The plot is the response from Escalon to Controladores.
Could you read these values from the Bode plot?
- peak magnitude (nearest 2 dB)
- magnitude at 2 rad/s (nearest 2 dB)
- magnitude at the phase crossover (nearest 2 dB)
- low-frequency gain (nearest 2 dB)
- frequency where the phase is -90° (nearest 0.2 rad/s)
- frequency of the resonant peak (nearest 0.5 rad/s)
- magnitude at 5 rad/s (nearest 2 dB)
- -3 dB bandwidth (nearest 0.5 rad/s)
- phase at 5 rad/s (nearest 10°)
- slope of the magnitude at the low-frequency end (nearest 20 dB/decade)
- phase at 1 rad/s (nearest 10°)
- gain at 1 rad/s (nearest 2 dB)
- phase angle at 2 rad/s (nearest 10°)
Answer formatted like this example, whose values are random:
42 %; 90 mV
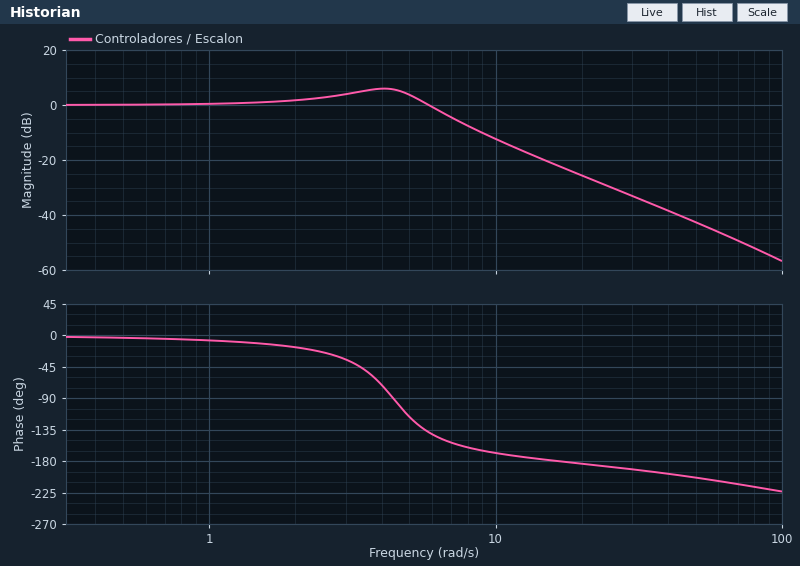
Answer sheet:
6 dB; 2 dB; -22 dB; 0 dB; 4.4 rad/s; 4.0 rad/s; 4 dB; 6.5 rad/s; -120°; 0 dB/decade; -10°; 0 dB; -20°
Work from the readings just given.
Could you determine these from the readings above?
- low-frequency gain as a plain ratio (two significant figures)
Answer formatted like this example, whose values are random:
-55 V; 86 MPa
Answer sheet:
1.0
